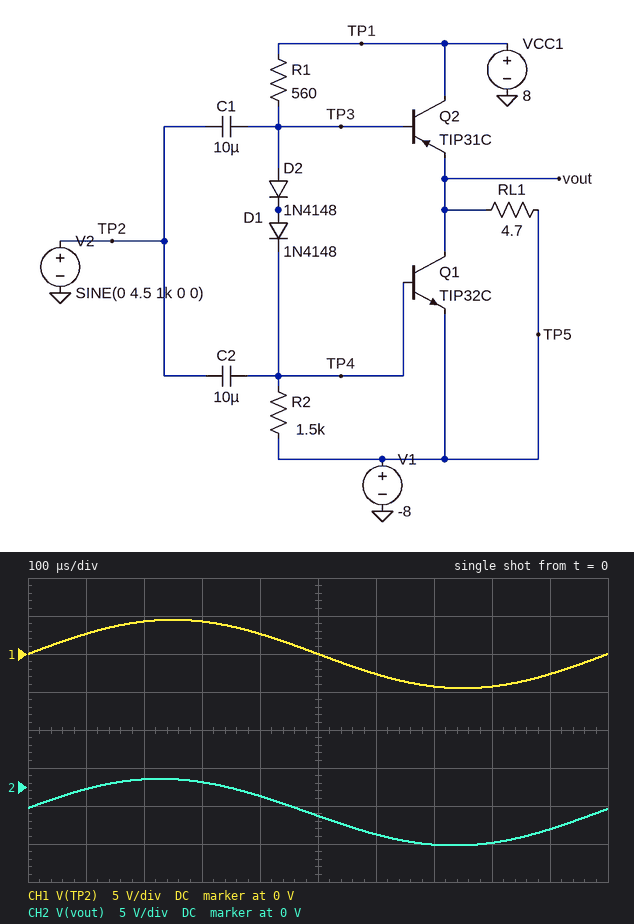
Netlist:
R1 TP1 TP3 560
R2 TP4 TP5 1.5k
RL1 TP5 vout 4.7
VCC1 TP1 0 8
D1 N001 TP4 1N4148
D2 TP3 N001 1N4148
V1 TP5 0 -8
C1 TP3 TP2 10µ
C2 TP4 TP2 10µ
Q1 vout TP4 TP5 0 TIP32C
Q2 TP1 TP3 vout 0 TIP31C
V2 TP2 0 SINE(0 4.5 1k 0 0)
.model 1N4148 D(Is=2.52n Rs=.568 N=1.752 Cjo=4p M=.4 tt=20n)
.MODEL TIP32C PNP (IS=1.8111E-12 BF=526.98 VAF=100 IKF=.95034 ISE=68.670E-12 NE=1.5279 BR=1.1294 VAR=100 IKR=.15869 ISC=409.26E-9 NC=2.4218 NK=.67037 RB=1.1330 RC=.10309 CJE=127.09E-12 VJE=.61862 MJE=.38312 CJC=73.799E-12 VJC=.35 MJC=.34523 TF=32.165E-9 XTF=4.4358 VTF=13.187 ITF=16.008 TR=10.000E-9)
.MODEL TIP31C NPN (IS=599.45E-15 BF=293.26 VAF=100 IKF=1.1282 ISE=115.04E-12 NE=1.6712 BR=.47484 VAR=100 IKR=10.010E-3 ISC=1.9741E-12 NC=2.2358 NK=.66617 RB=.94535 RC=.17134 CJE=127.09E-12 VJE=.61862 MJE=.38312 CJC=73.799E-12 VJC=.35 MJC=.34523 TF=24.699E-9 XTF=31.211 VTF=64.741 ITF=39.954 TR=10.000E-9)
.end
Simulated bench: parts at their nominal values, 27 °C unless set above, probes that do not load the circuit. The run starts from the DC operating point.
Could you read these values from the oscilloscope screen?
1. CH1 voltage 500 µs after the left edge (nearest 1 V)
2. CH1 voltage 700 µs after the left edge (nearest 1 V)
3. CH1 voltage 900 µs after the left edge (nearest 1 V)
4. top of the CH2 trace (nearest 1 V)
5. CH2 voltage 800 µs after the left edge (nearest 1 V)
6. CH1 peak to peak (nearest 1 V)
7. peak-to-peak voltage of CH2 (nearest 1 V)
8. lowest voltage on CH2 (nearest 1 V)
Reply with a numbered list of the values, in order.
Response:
1. 0 V
2. -4 V
3. -3 V
4. 1 V
5. -7 V
6. 9 V
7. 9 V
8. -8 V
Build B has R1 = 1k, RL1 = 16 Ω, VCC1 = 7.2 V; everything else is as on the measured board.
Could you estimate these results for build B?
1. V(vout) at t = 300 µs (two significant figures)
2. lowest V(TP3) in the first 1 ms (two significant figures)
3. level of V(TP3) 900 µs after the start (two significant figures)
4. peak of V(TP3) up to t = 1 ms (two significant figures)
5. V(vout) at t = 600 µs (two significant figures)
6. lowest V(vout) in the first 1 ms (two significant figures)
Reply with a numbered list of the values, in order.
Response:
1. 3.7 V
2. -4.3 V
3. -2.3 V
4. 4.7 V
5. -3.2 V
6. -5.0 V
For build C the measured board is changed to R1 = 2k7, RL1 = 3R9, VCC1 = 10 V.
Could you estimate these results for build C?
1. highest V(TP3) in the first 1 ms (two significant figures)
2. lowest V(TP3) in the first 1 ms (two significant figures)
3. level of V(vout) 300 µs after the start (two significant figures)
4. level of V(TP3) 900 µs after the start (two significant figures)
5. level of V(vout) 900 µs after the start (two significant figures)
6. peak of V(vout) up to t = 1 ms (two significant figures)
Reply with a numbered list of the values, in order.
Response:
1. -1.0 V
2. -10 V
3. -2.2 V
4. -8.2 V
5. -8.0 V
6. -1.8 V
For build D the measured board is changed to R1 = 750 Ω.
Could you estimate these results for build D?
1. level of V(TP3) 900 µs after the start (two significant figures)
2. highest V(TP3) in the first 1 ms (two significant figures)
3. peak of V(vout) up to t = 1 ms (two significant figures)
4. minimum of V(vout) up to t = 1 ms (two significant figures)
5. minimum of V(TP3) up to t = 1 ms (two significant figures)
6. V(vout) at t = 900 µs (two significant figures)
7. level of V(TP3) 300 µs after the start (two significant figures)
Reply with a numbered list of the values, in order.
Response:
1. -5.5 V
2. 1.3 V
3. 510 mV
4. -8.0 V
5. -7.7 V
6. -6.2 V
7. 920 mV
